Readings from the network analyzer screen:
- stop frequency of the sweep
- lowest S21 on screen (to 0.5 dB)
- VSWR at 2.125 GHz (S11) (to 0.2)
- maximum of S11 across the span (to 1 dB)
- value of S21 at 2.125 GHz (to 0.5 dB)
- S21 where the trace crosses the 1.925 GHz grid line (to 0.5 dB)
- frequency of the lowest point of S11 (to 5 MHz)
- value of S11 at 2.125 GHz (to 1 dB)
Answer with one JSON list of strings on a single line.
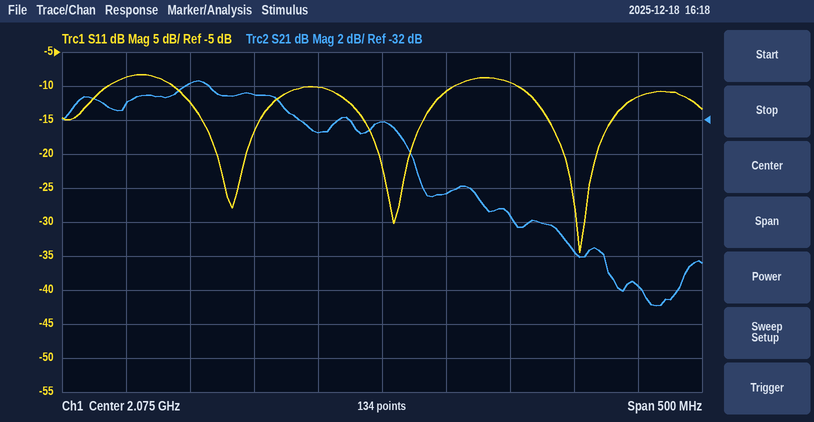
["2.325 GHz", "-43.0 dB", "1.8", "-8 dB", "-36.5 dB", "-30.0 dB", "2.230 GHz", "-11 dB"]
